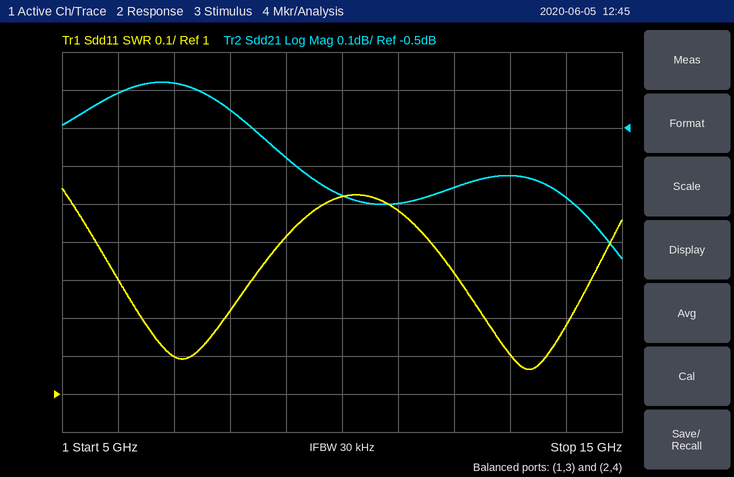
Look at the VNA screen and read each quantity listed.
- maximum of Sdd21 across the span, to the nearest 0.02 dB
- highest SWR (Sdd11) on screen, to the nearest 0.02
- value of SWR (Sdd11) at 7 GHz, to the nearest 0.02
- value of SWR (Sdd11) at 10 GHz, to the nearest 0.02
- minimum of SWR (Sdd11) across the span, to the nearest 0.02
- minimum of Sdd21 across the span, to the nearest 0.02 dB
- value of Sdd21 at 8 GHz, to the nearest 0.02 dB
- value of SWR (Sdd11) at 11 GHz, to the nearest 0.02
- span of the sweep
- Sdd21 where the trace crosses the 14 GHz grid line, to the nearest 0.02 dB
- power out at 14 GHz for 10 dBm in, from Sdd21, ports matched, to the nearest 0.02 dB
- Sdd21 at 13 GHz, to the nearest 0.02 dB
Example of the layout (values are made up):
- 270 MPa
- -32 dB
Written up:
- -0.38 dB
- 1.54
- 1.10
- 1.52
- 1.06
- -0.84 dB
- -0.46 dB
- 1.48
- 10 GHz
- -0.68 dB
- 9.32 dBm
- -0.62 dB
